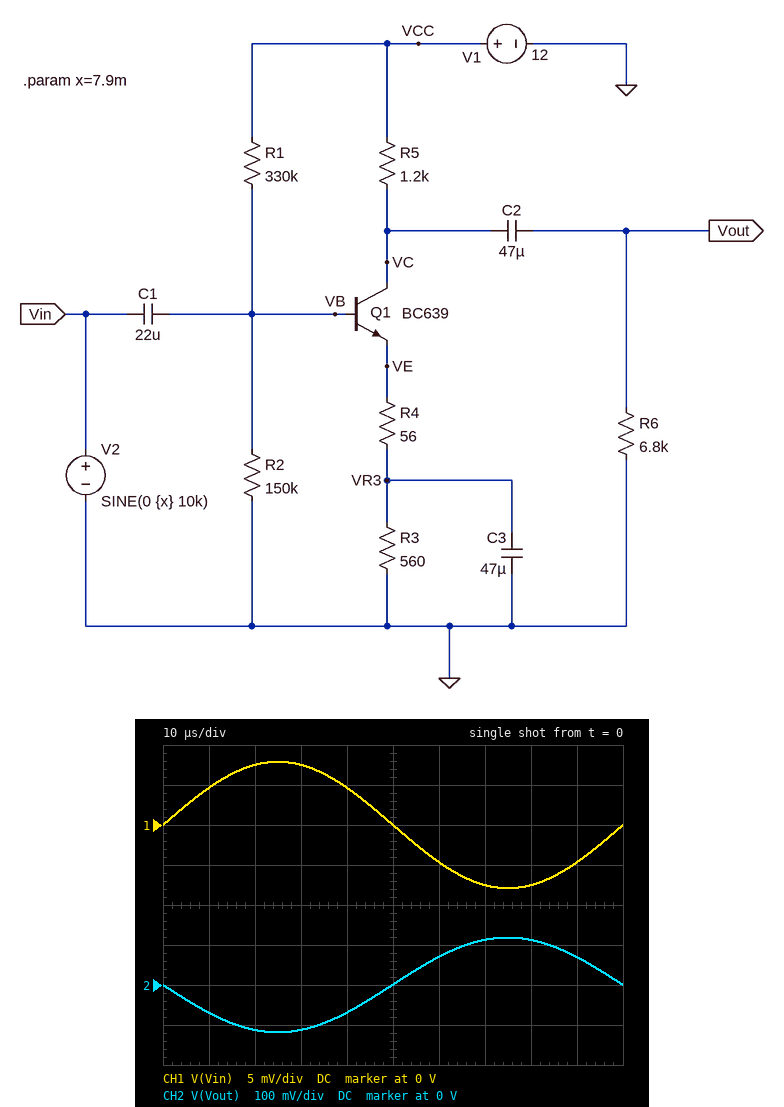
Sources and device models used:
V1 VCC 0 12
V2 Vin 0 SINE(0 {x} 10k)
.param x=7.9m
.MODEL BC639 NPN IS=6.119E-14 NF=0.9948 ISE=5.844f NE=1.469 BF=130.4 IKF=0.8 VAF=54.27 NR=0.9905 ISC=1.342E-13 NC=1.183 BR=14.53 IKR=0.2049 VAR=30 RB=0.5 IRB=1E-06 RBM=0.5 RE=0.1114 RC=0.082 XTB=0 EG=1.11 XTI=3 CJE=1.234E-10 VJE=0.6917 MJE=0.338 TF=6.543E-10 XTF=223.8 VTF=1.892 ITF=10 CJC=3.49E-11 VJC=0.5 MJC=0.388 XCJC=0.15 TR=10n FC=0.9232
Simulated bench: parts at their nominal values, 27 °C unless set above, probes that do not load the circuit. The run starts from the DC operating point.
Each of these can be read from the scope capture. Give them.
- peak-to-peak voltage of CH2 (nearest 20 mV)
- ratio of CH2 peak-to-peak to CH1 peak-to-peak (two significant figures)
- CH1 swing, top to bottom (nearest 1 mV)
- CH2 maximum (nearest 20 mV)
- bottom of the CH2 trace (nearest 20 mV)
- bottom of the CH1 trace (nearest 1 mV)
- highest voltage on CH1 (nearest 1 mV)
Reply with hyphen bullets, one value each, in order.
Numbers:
- 240 mV
- 15
- 16 mV
- 120 mV
- -120 mV
- -8 mV
- 8 mV
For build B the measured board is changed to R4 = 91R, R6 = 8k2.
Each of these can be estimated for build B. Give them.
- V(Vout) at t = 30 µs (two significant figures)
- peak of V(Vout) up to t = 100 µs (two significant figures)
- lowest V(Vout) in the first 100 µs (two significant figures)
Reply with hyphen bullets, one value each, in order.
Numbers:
- -76 mV
- 80 mV
- -80 mV
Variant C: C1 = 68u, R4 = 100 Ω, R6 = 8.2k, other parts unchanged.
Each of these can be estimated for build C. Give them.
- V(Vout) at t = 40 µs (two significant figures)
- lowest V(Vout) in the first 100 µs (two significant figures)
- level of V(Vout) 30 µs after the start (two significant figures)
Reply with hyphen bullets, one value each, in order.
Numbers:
- -43 mV
- -73 mV
- -70 mV
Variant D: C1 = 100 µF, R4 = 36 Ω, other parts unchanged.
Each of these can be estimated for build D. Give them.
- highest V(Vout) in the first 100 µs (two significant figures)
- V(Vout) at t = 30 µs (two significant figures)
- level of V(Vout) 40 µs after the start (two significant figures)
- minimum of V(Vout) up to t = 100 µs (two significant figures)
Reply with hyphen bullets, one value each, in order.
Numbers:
- 170 mV
- -160 mV
- -98 mV
- -170 mV
